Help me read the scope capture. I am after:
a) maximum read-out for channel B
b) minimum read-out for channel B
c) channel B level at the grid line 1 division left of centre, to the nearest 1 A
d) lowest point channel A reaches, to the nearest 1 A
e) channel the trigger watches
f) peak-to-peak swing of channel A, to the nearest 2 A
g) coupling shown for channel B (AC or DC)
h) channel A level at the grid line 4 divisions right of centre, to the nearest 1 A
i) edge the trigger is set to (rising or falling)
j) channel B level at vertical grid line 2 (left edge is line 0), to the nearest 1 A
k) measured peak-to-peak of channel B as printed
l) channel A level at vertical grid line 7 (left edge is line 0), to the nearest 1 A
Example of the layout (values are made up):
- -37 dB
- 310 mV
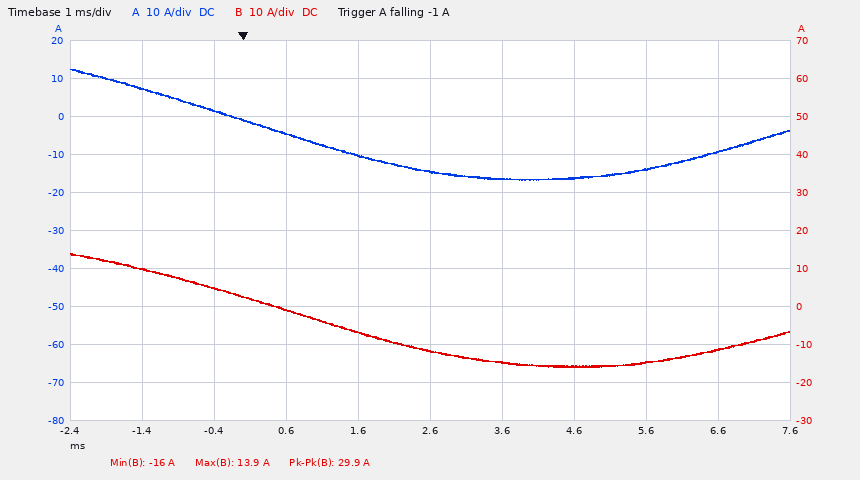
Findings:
- 13.9 A
- -16 A
- -7 A
- -17 A
- channel A
- 30 A
- DC
- -9 A
- falling
- 5 A
- 29.9 A
- -16 A
